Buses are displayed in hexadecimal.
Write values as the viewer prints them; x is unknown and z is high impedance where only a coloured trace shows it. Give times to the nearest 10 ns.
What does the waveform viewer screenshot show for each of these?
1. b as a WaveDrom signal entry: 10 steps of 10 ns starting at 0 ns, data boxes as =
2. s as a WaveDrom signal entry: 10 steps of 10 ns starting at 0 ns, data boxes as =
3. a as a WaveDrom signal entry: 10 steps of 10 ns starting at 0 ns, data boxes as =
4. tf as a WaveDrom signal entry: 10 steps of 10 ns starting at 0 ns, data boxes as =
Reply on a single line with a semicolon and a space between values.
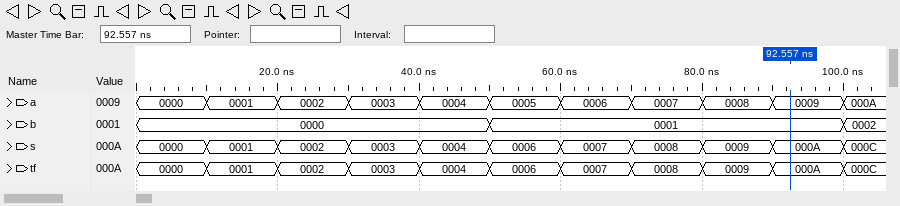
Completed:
{name: 'b', wave: '=....=....', data: '0000 0001'}; {name: 's', wave: '==========', data: '0000 0001 0002 0003 0004 0006 0007 0008 0009 000A'}; {name: 'a', wave: '==========', data: '0000 0001 0002 0003 0004 0005 0006 0007 0008 0009'}; {name: 'tf', wave: '==========', data: '0000 0001 0002 0003 0004 0006 0007 0008 0009 000A'}
